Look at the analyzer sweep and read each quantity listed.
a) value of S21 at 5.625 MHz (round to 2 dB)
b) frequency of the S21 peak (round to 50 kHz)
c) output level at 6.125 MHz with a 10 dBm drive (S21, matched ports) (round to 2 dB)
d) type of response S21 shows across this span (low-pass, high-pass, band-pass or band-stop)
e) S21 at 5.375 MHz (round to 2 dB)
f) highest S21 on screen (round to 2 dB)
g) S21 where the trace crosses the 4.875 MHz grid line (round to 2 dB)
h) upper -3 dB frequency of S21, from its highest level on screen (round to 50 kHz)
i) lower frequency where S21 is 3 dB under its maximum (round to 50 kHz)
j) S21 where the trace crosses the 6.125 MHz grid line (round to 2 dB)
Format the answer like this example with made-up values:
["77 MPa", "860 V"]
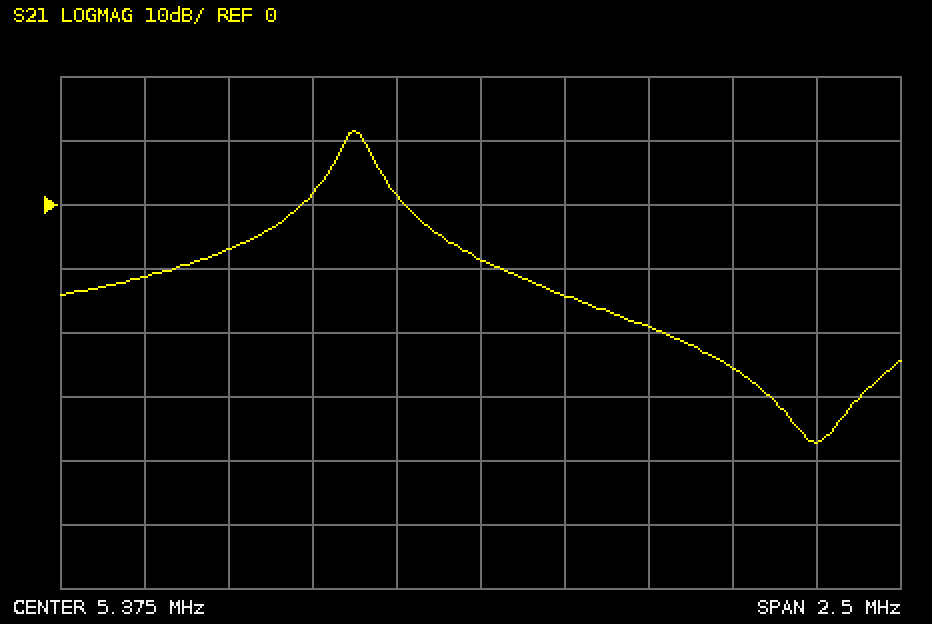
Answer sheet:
["-14 dB", "5.00 MHz", "-16 dBm", "band-pass", "-8 dB", "12 dB", "2 dB", "5.05 MHz", "4.95 MHz", "-26 dB"]
